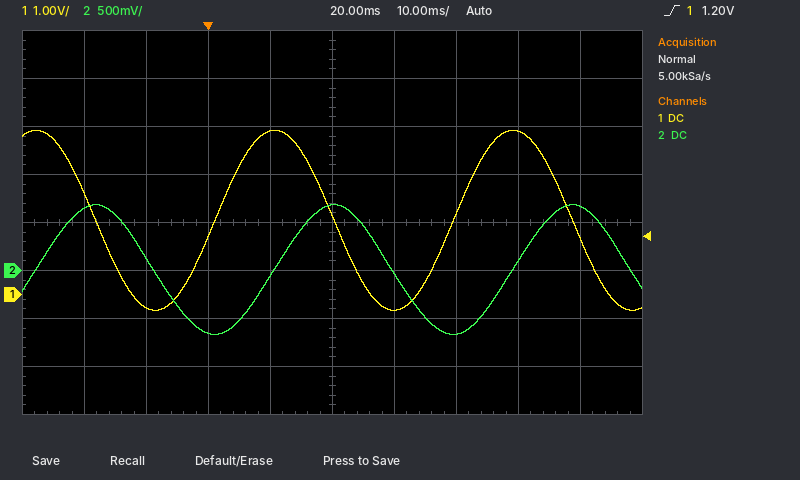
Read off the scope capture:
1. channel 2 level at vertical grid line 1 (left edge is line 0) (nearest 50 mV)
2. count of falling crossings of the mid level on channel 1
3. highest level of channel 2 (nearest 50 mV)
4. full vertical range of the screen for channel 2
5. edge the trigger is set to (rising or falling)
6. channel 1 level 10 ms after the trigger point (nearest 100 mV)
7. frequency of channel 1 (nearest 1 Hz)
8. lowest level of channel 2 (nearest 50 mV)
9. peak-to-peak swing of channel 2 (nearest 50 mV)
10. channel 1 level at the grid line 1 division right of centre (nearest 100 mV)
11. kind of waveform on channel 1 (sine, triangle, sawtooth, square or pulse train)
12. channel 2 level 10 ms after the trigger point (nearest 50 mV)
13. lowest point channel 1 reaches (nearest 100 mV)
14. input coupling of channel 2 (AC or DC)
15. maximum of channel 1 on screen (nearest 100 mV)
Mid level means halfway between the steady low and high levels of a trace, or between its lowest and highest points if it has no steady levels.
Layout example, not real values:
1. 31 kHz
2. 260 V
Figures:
1. 650 mV
2. 3
3. 700 mV
4. 4 V
5. rising
6. 3.4 V
7. 26 Hz
8. -650 mV
9. 1.35 V
10. -300 mV
11. sine
12. -50 mV
13. -300 mV
14. DC
15. 3.4 V
